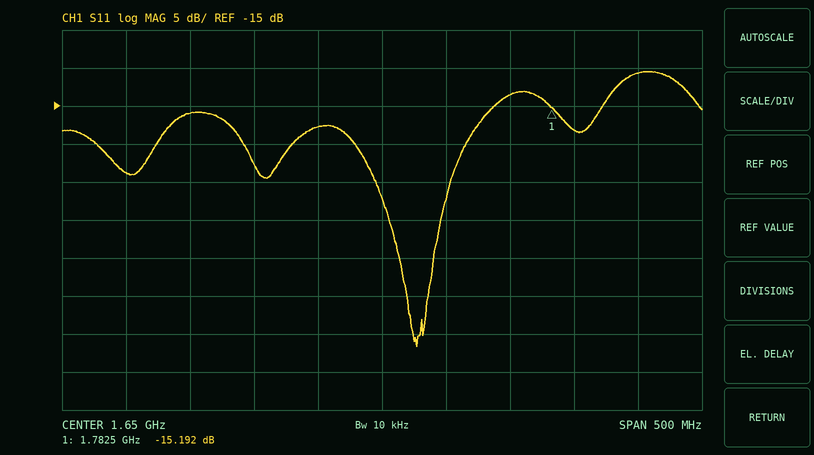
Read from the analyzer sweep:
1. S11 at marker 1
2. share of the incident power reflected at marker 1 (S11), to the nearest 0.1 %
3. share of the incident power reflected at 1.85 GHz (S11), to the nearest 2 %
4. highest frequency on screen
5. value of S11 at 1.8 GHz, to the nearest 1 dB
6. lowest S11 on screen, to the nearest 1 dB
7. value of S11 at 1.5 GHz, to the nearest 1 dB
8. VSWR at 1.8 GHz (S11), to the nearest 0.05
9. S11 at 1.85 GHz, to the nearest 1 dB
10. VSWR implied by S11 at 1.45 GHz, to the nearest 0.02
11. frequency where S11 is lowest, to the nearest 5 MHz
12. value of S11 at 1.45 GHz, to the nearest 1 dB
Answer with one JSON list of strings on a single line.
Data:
["-15.192 dB", "3.0 %", "8 %", "1.9 GHz", "-18 dB", "-47 dB", "-16 dB", "1.30", "-11 dB", "1.14", "1.675 GHz", "-24 dB"]
